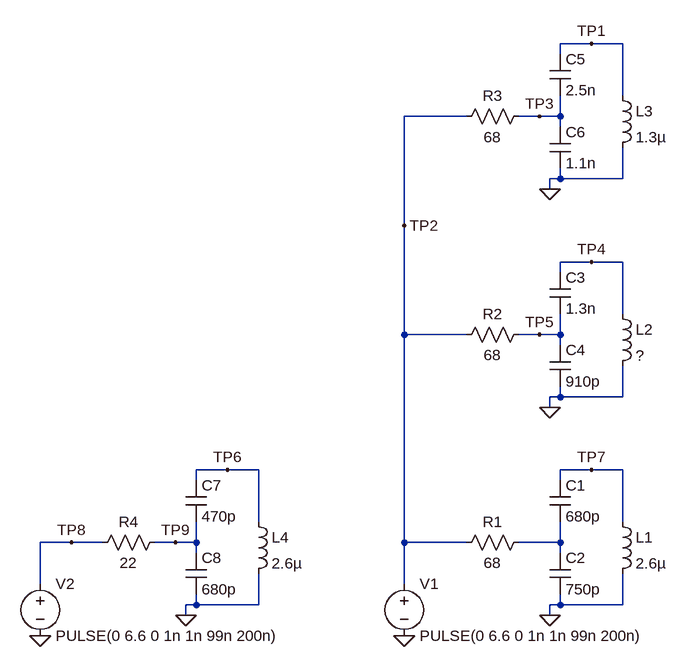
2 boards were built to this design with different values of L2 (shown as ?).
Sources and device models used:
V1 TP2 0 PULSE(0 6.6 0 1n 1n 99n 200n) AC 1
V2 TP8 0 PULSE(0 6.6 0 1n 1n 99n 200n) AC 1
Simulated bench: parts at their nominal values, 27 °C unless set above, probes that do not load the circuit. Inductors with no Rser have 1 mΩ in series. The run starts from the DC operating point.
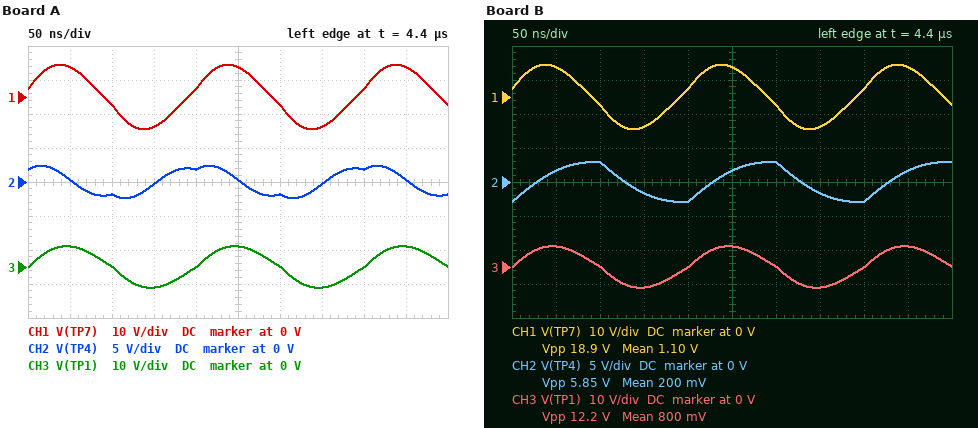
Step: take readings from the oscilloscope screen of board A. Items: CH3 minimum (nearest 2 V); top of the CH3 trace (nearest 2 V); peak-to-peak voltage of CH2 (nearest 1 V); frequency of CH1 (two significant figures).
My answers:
-6 V
6 V
5 V
5.0 MHz
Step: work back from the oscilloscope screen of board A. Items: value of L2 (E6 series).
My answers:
1 µH
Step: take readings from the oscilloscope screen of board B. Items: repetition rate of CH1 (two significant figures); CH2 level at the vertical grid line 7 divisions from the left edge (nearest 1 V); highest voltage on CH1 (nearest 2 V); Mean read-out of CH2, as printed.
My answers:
5.0 MHz
-2 V
10 V
200 mV
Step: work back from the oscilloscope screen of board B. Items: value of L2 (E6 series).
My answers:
4.7 µH
